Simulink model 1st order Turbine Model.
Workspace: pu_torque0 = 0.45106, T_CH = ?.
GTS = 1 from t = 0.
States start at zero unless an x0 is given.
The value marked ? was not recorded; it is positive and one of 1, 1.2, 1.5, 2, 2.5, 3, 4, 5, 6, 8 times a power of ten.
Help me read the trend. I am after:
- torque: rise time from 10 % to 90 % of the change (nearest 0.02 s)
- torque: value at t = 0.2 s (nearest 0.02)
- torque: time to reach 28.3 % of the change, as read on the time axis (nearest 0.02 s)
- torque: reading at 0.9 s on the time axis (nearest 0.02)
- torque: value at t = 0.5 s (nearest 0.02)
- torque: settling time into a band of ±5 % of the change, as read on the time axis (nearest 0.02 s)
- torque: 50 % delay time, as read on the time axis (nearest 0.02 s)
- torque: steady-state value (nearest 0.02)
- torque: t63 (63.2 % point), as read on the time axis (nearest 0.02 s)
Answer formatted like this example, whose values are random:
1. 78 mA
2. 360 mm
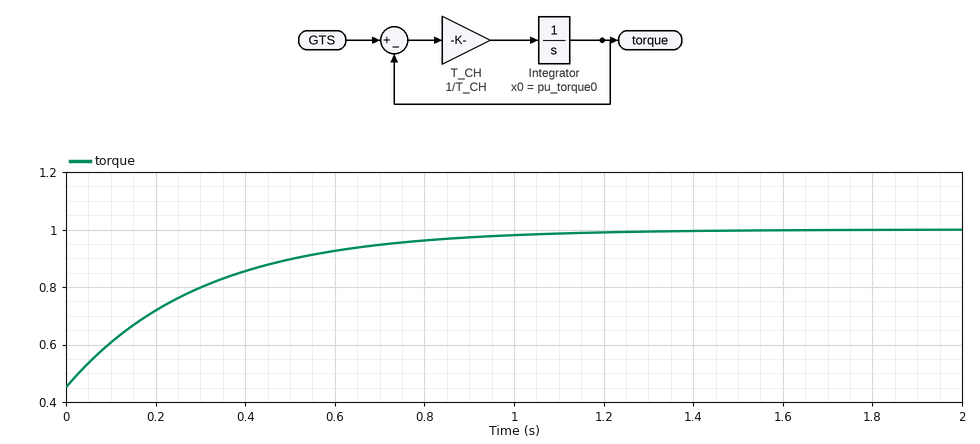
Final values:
1. 0.66 s
2. 0.72
3. 0.10 s
4. 0.98
5. 0.90
6. 0.90 s
7. 0.20 s
8. 1.00
9. 0.30 s
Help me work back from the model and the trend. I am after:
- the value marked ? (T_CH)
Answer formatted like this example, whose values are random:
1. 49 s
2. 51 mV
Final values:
1. 0.3
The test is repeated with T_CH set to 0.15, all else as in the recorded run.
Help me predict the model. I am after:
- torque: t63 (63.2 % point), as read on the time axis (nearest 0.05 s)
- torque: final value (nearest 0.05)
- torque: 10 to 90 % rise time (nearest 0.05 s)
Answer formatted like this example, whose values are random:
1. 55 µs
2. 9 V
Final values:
1. 0.15 s
2. 1.00
3. 0.35 s
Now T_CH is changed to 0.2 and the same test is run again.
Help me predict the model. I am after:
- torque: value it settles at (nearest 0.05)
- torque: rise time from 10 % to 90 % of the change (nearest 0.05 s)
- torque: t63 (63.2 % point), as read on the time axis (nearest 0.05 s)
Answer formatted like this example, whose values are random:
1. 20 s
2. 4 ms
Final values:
1. 1.00
2. 0.45 s
3. 0.20 s
